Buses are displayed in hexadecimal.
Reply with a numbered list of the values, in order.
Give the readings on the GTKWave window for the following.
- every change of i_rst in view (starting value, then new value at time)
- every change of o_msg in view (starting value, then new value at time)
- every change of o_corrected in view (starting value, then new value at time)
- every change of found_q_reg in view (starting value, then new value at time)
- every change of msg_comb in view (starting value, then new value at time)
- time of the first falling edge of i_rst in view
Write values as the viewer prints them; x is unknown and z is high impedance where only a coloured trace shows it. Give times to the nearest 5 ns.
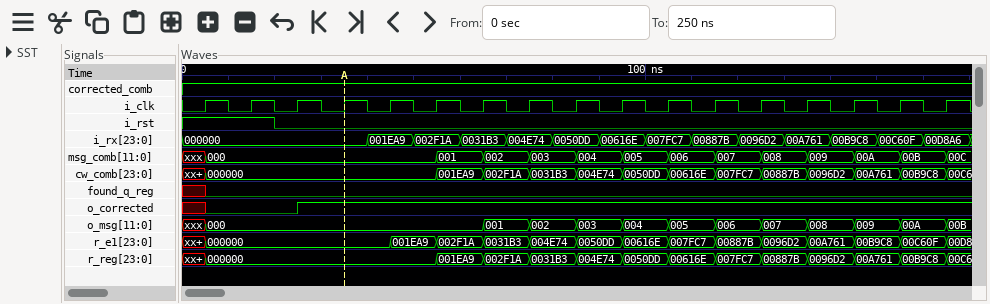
1. 1, 0 at 20 ns
2. xxx, 000 at 5 ns, 001 at 65 ns, 002 at 75 ns, 003 at 85 ns, 004 at 95 ns, 005 at 105 ns, 006 at 115 ns, 007 at 125 ns, 008 at 135 ns, 009 at 145 ns, 00A at 155 ns, 00B at 165 ns
3. x, 0 at 5 ns, 1 at 25 ns
4. x, 0 at 5 ns
5. xxx, 000 at 5 ns, 001 at 55 ns, 002 at 65 ns, 003 at 75 ns, 004 at 85 ns, 005 at 95 ns, 006 at 105 ns, 007 at 115 ns, 008 at 125 ns, 009 at 135 ns, 00A at 145 ns, 00B at 155 ns, 00C at 165 ns
6. 20 ns
